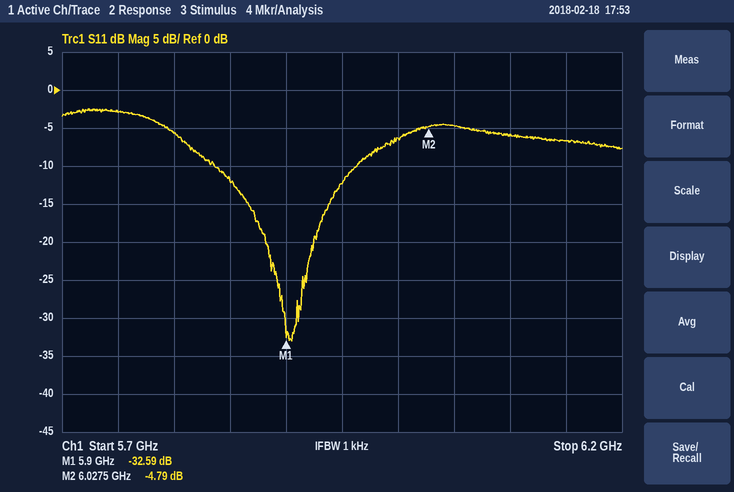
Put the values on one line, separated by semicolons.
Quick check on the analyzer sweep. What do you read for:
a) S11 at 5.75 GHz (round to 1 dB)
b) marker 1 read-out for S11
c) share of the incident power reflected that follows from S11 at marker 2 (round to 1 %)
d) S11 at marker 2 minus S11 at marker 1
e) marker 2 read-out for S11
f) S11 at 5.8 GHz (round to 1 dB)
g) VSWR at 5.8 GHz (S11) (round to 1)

-3 dB; -32.59 dB; 33 %; 27.80 dB; -4.79 dB; -6 dB; 3
